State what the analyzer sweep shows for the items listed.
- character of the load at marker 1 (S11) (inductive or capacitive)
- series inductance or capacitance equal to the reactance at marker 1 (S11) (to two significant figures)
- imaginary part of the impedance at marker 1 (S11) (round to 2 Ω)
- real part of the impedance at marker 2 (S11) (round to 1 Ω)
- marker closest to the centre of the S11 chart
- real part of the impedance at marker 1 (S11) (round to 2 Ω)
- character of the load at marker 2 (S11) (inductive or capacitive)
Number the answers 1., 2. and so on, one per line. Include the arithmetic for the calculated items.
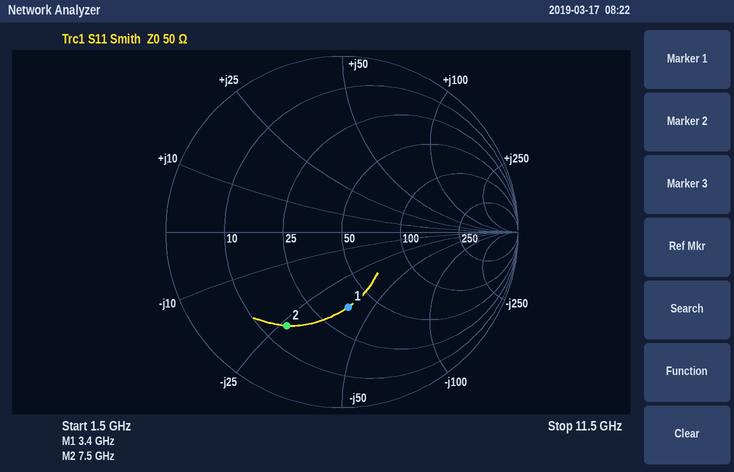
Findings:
1. capacitive
2. C = 1/(2π × 3.4 GHz × 38 Ω) ≈ 1.2 pF
3. -38 Ω
4. 15 Ω
5. marker 1
6. 36 Ω
7. capacitive
